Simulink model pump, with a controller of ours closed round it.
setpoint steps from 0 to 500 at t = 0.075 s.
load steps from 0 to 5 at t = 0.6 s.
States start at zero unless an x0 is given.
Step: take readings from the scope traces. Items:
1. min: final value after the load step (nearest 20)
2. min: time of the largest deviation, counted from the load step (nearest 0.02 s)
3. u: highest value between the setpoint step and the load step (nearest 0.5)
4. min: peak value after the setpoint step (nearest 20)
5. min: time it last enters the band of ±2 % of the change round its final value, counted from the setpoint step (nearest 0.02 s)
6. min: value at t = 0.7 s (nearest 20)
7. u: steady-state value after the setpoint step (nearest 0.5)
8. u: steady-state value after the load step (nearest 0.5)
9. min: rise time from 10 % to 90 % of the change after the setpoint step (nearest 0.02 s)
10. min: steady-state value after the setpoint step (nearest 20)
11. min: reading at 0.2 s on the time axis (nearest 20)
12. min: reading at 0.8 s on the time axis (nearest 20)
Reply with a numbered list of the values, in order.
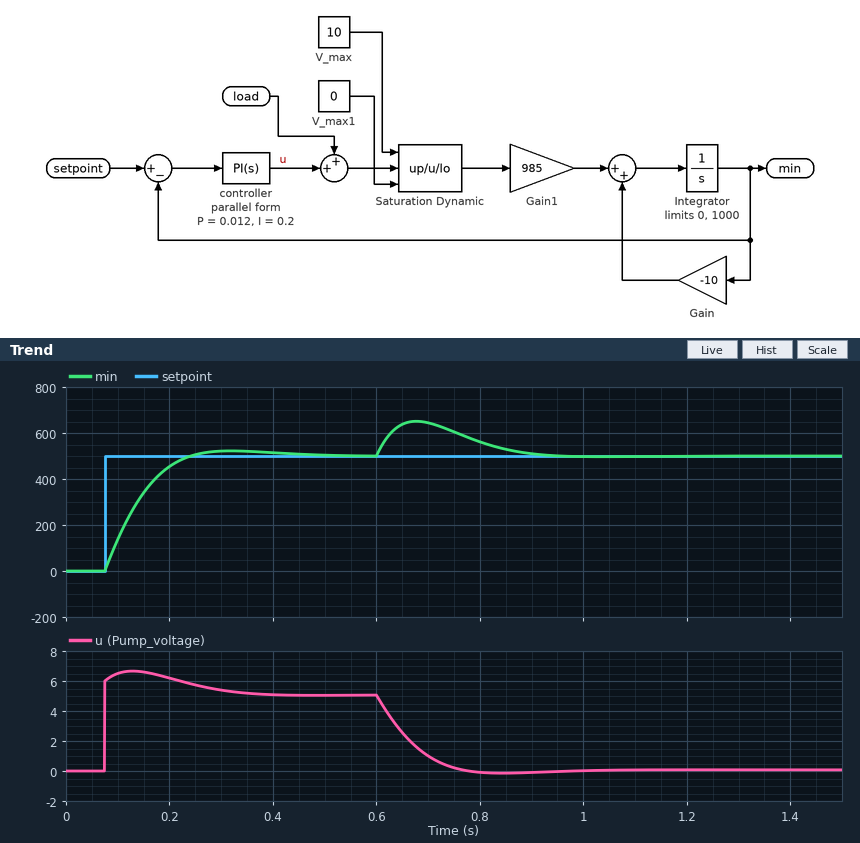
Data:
1. 500
2. 0.08 s
3. 6.5
4. 520
5. 0.36 s
6. 640
7. 5.0
8. 0.0
9. 0.12 s
10. 500
11. 460
12. 560
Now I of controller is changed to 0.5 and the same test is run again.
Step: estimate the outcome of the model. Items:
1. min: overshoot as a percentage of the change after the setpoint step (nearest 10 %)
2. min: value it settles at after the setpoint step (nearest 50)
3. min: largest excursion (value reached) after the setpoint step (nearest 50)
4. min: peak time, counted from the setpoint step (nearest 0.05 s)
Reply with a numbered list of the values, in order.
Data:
1. 20 %
2. 500
3. 600
4. 0.15 s
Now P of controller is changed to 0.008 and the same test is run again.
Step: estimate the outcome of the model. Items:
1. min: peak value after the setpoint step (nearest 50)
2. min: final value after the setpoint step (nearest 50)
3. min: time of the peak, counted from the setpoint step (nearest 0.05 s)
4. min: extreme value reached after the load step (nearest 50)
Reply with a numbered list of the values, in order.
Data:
1. 550
2. 500
3. 0.25 s
4. 650
